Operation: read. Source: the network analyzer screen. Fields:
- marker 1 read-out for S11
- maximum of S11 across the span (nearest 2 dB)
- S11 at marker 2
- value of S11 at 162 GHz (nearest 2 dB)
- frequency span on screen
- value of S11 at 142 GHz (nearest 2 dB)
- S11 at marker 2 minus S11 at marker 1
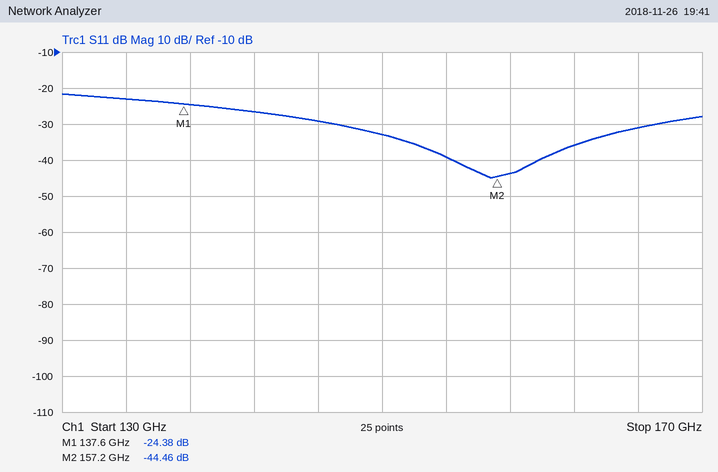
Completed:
-24.38 dB
-22 dB
-44.46 dB
-36 dB
40 GHz
-26 dB
-20.08 dB
